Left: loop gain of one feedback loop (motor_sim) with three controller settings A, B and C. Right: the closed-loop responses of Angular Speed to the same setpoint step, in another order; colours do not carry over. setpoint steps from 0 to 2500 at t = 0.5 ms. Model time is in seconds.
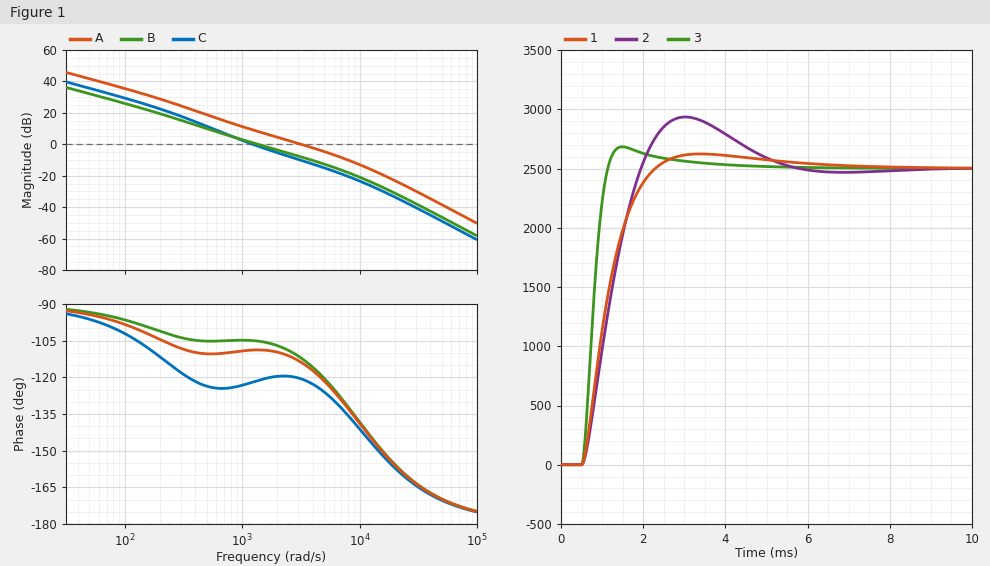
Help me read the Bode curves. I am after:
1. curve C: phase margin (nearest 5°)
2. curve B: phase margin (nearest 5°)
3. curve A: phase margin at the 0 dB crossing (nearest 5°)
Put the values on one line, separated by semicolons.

60°; 75°; 65°
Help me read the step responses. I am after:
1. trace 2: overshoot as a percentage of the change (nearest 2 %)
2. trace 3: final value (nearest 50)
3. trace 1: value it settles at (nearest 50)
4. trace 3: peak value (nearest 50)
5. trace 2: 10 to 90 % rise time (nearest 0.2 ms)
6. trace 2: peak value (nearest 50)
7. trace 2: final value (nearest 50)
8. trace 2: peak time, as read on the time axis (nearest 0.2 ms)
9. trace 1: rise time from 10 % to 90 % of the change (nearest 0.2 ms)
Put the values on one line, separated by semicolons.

18 %; 2500; 2500; 2700; 1.0 ms; 2950; 2500; 3.0 ms; 1.2 ms
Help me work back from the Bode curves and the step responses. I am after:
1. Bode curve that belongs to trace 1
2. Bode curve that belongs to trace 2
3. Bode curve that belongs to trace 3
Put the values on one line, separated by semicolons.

B; C; A
